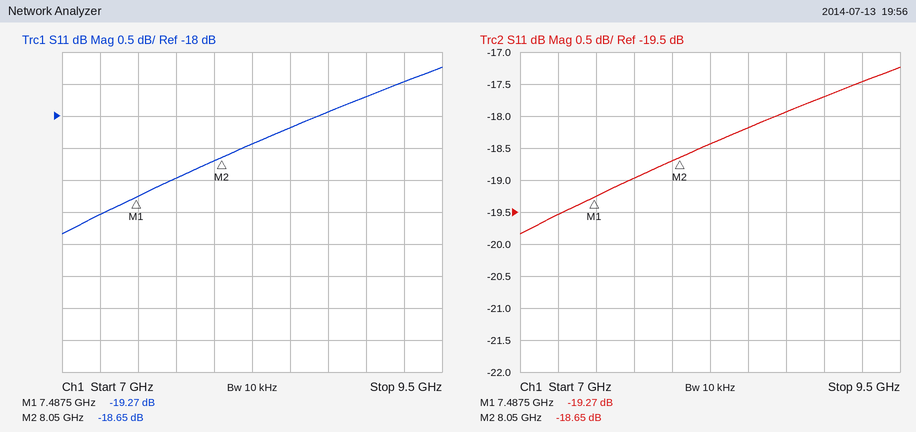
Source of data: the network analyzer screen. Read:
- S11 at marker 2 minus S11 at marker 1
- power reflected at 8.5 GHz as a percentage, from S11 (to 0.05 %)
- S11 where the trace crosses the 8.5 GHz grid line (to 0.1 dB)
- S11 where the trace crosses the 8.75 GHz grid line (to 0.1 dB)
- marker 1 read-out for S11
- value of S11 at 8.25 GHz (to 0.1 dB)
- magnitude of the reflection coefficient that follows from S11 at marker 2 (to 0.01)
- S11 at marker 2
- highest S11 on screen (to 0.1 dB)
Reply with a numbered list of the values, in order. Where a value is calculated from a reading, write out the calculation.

1. -18.65 − (-19.27) = 0.62 dB
2. 10^(-18.2/10) ≈ 1.51 %, so 1.50 % to the nearest 0.05 %
3. -18.2 dB
4. -17.9 dB
5. -19.27 dB
6. -18.4 dB
7. 10^(-18.65/20) ≈ 0.12
8. -18.65 dB
9. -17.2 dB
